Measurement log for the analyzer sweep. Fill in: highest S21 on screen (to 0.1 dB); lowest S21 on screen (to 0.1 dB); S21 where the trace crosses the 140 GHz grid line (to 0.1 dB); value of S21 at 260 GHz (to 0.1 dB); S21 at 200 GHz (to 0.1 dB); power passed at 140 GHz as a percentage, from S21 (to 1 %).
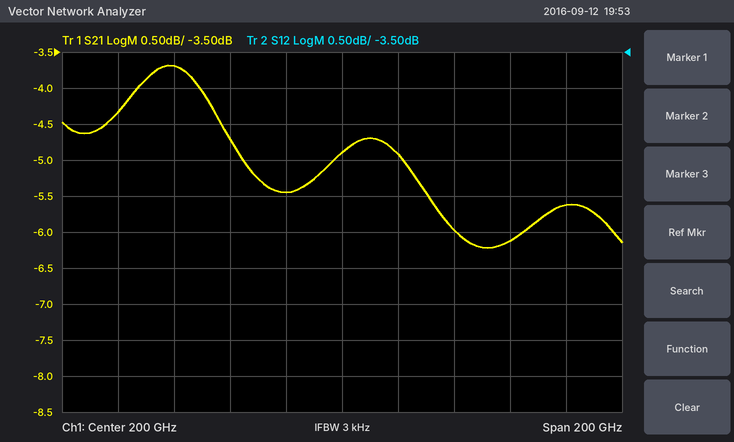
-3.7 dB
-6.2 dB
-3.7 dB
-6.1 dB
-4.9 dB
43 %
